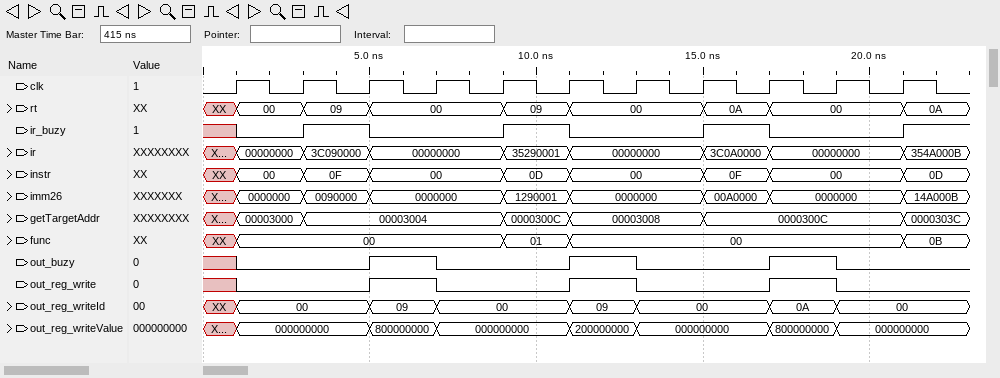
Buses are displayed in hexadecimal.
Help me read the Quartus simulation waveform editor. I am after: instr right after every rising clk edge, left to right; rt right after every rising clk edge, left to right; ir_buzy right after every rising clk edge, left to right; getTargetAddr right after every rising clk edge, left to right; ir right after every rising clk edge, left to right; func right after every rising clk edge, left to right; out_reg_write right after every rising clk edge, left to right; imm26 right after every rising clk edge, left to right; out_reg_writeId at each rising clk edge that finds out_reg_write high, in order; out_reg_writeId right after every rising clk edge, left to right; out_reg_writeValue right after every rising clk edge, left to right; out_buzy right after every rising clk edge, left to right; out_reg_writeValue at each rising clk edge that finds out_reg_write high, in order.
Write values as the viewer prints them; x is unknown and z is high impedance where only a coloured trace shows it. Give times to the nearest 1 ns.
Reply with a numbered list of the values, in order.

1. 00, 0F, 00, 00, 0D, 00, 00, 0F, 00, 00, 0D
2. 00, 09, 00, 00, 09, 00, 00, 0A, 00, 00, 0A
3. 0 1 0 0 1 0 0 1 0 0 1
4. 00003000, 00003004, 00003004, 00003004, 0000300C, 00003008, 00003008, 0000300C, 0000300C, 0000300C, 0000303C
5. 00000000, 3C090000, 00000000, 00000000, 35290001, 00000000, 00000000, 3C0A0000, 00000000, 00000000, 354A000B
6. 00, 00, 00, 00, 01, 00, 00, 00, 00, 00, 0B
7. 0 0 1 0 0 1 0 0 1 0 0
8. 0000000, 0090000, 0000000, 0000000, 1290001, 0000000, 0000000, 00A0000, 0000000, 0000000, 14A000B
9. 09, 09, 0A
10. 00, 00, 09, 00, 00, 09, 00, 00, 0A, 00, 00
11. 000000000, 000000000, 800000000, 000000000, 000000000, 200000000, 000000000, 000000000, 800000000, 000000000, 000000000
12. 0 0 1 0 0 1 0 0 1 0 0
13. 800000000, 200000000, 800000000
